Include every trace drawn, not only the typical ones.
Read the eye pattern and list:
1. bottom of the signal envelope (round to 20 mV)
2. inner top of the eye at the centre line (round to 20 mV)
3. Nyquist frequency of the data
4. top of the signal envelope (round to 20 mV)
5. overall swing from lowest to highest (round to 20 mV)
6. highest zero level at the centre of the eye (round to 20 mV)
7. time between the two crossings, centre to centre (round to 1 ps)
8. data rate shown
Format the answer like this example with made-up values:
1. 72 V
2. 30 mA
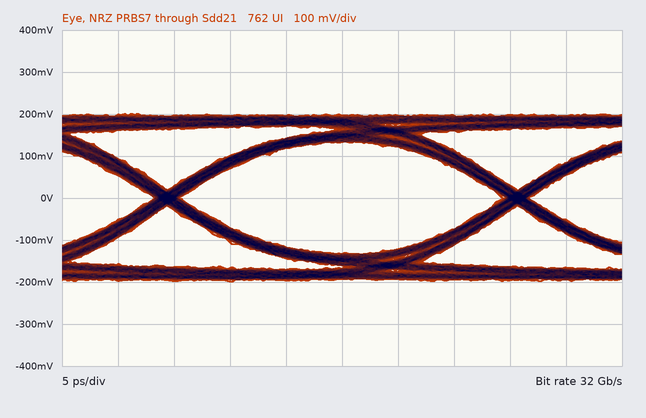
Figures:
1. -200 mV
2. 140 mV
3. 16 GHz
4. 200 mV
5. 400 mV
6. -140 mV
7. 31 ps
8. 32 Gb/s
